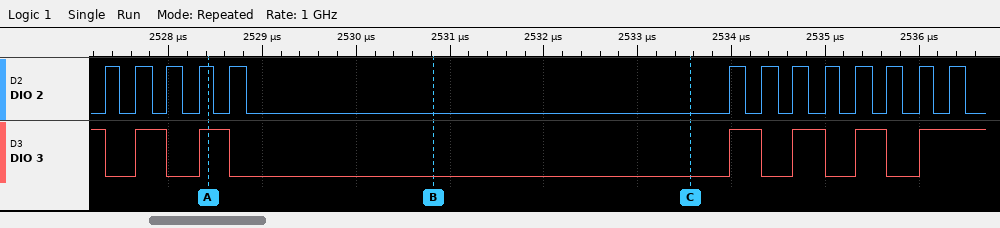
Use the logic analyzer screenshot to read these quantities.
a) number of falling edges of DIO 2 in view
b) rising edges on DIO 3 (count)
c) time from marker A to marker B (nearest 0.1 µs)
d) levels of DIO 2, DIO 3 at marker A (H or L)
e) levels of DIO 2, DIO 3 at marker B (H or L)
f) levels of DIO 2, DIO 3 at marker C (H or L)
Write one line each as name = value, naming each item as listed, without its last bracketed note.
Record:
number of falling edges of DIO 2 in view = 13
rising edges on DIO 3 = 6
time from marker A to marker B = 2.4 µs
levels of DIO 2, DIO 3 at marker A = DIO 2=H, DIO 3=H
levels of DIO 2, DIO 3 at marker B = DIO 2=L, DIO 3=L
levels of DIO 2, DIO 3 at marker C = DIO 2=L, DIO 3=L
